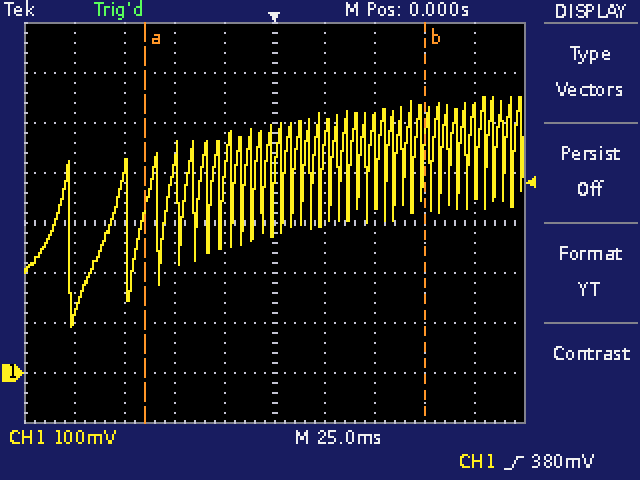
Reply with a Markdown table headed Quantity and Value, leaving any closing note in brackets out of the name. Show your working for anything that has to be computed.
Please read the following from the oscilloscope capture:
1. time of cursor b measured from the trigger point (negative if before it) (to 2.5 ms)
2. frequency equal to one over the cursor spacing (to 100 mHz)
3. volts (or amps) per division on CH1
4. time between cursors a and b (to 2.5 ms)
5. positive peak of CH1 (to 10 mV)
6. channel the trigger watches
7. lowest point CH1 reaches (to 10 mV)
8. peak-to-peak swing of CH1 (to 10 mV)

| Quantity | Value |
|---|---|
| time of cursor b measured from the trigger point (negative if before it) | +75.0 ms |
| frequency equal to one over the cursor spacing | 1 / 140.0 ms ≈ 7.1 Hz |
| volts (or amps) per division on CH1 | 100 mV |
| time between cursors a and b | 140.0 ms |
| positive peak of CH1 | 550 mV |
| channel the trigger watches | CH1 |
| lowest point CH1 reaches | 90 mV |
| peak-to-peak swing of CH1 | 550 mV − (90 mV) = 460 mV |
